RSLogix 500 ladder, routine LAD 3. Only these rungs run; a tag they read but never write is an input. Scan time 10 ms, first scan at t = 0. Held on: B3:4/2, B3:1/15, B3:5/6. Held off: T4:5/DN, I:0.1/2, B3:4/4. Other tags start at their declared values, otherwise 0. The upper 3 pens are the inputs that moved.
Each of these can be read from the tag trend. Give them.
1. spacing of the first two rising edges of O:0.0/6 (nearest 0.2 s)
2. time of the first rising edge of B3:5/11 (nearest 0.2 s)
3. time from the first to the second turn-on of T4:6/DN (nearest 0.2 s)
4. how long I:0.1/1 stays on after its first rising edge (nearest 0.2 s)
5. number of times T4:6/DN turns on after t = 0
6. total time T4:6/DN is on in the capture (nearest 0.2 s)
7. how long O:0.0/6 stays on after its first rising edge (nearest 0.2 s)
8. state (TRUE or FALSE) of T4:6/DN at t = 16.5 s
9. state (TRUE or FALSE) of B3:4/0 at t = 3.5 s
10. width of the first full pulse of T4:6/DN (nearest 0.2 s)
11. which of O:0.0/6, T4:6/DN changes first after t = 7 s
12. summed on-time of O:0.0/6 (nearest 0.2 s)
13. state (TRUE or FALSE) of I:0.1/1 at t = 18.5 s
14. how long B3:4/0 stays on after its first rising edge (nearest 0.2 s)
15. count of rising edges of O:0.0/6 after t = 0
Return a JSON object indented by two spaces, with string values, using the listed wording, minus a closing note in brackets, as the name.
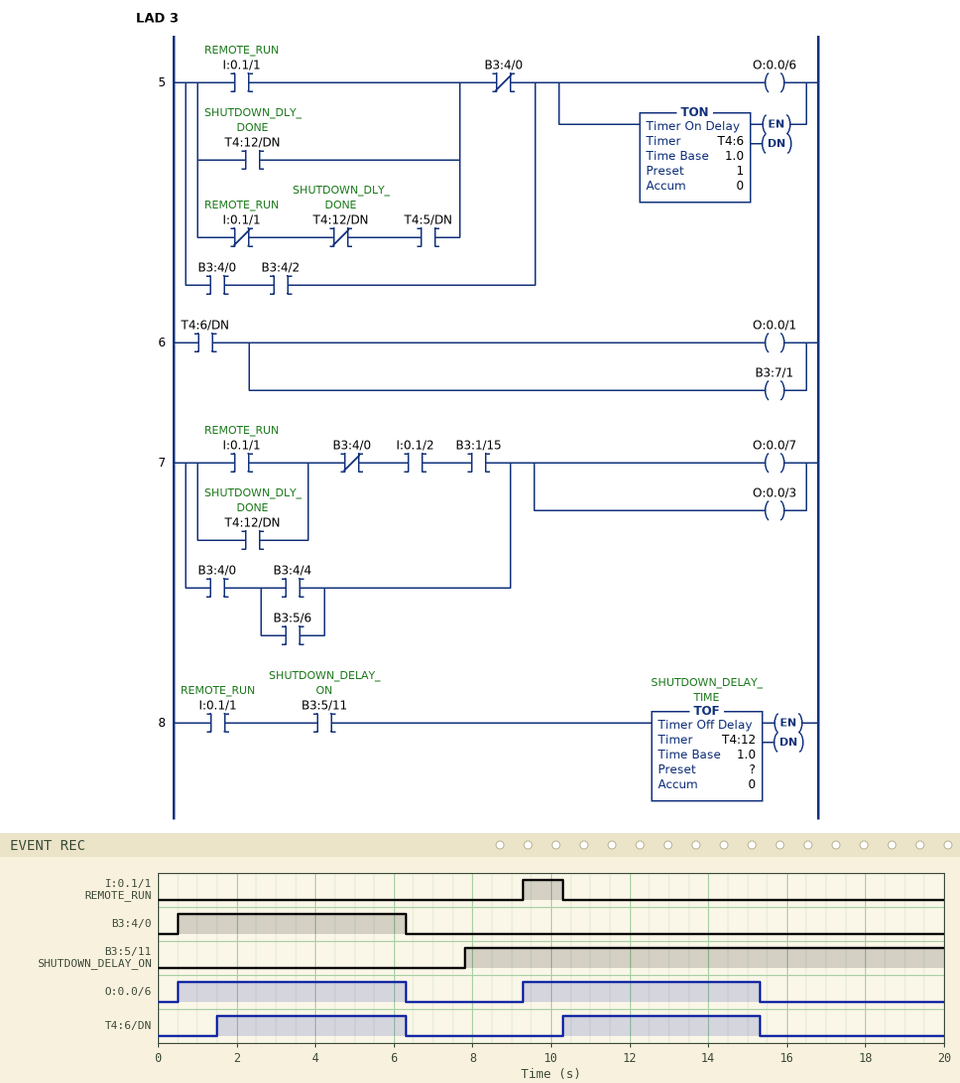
{
  "spacing of the first two rising edges of O:0.0/6": "8.8 s",
  "time of the first rising edge of B3:5/11": "7.8 s",
  "time from the first to the second turn-on of T4:6/DN": "8.8 s",
  "how long I:0.1/1 stays on after its first rising edge": "1.0 s",
  "number of times T4:6/DN turns on after t = 0": "2",
  "total time T4:6/DN is on in the capture": "9.8 s",
  "how long O:0.0/6 stays on after its first rising edge": "5.8 s",
  "state (TRUE or FALSE) of T4:6/DN at t = 16.5 s": "FALSE",
  "state (TRUE or FALSE) of B3:4/0 at t = 3.5 s": "TRUE",
  "width of the first full pulse of T4:6/DN": "4.8 s",
  "which of O:0.0/6, T4:6/DN changes first after t = 7 s": "O:0.0/6",
  "summed on-time of O:0.0/6": "11.8 s",
  "state (TRUE or FALSE) of I:0.1/1 at t = 18.5 s": "FALSE",
  "how long B3:4/0 stays on after its first rising edge": "5.8 s",
  "count of rising edges of O:0.0/6 after t = 0": "2"
}
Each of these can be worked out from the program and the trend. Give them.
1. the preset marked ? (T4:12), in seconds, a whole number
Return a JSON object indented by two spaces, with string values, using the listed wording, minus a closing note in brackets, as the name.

{
  "the preset marked ? (T4:12), in seconds, a whole number": "5 s"
}
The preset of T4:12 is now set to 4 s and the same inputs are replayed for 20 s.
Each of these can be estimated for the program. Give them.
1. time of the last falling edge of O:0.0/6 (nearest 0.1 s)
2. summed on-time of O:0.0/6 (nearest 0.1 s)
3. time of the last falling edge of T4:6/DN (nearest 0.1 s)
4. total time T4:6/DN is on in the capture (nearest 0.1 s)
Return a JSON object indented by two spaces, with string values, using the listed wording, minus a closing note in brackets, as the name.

{
  "time of the last falling edge of O:0.0/6": "14.3 s",
  "summed on-time of O:0.0/6": "10.8 s",
  "time of the last falling edge of T4:6/DN": "14.3 s",
  "total time T4:6/DN is on in the capture": "8.8 s"
}
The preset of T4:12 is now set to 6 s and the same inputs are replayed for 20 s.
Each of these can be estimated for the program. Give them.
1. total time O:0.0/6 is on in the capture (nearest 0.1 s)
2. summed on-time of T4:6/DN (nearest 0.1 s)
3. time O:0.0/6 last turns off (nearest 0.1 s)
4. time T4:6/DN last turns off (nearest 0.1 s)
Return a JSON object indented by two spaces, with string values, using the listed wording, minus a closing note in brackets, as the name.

{
  "total time O:0.0/6 is on in the capture": "12.8 s",
  "summed on-time of T4:6/DN": "10.8 s",
  "time O:0.0/6 last turns off": "16.3 s",
  "time T4:6/DN last turns off": "16.3 s"
}
